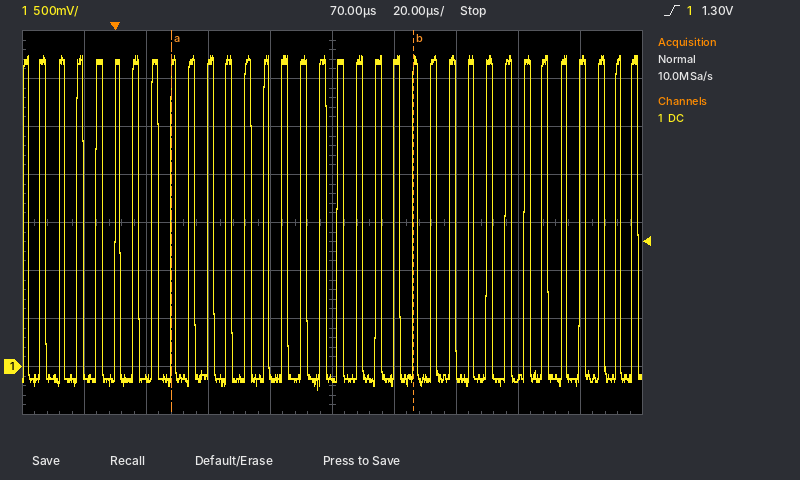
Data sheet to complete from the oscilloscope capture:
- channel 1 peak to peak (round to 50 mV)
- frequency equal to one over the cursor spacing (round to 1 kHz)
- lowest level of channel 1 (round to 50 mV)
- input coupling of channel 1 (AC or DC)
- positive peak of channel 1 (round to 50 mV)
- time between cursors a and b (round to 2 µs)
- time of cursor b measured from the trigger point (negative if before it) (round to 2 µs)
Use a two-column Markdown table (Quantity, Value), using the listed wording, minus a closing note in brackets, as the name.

| Quantity | Value |
|---|---|
| channel 1 peak to peak | 3.50 V |
| frequency equal to one over the cursor spacing | 13 kHz |
| lowest level of channel 1 | -250 mV |
| input coupling of channel 1 | DC |
| positive peak of channel 1 | 3.25 V |
| time between cursors a and b | 78 µs |
| time of cursor b measured from the trigger point (negative if before it) | +96 µs |
